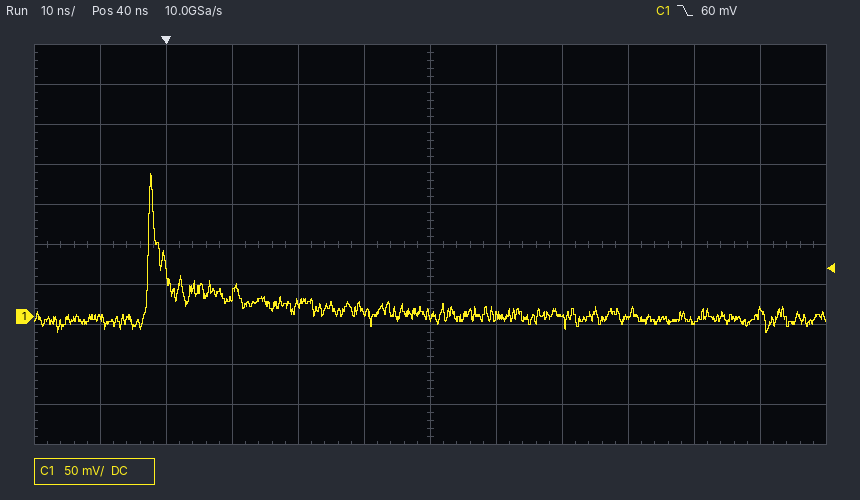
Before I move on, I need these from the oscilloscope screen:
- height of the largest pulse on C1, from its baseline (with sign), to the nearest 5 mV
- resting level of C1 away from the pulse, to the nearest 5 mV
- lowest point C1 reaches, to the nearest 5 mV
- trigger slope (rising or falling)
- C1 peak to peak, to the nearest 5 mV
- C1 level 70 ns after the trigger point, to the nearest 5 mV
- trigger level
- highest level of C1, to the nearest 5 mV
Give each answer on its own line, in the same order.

+180 mV
0 mV
-20 mV
falling
200 mV
0 mV
60 mV
180 mV
